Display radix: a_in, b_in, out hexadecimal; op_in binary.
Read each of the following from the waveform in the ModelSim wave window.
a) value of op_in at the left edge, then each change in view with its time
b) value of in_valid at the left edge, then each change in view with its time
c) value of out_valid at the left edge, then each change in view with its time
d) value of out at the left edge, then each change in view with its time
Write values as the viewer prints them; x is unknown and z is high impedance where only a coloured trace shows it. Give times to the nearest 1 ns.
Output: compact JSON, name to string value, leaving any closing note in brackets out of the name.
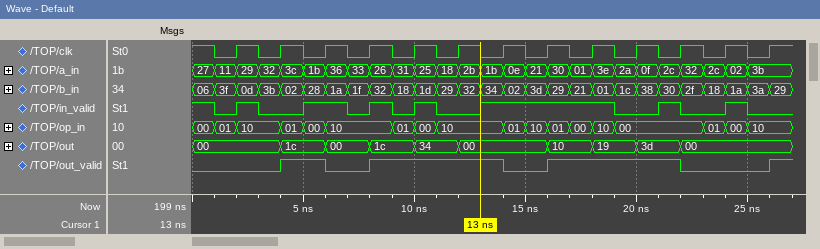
{"value of op_in at the left edge, then each change in view with its time": "00, 01 at 1 ns, 10 at 2 ns, 01 at 4 ns, 00 at 5 ns, 10 at 6 ns, 01 at 9 ns, 00 at 10 ns, 10 at 11 ns, 01 at 14 ns, 10 at 15 ns, 01 at 16 ns, 00 at 17 ns, 10 at 18 ns, 00 at 19 ns, 01 at 23 ns, 00 at 24 ns, 10 at 25 ns", "value of in_valid at the left edge, then each change in view with its time": "1, 0 at 1 ns, 1 at 2 ns, 0 at 3 ns, 1 at 5 ns, 0 at 7 ns, 1 at 8 ns, 0 at 9 ns, 1 at 10 ns, 0 at 11 ns, 1 at 13 ns, 0 at 19 ns, 1 at 21 ns, 0 at 22 ns, 1 at 24 ns, 0 at 25 ns", "value of out_valid at the left edge, then each change in view with its time": "0, 1 at 4 ns, 0 at 6 ns, 1 at 8 ns, 0 at 14 ns, 1 at 16 ns, 0 at 22 ns, 1 at 26 ns", "value of out at the left edge, then each change in view with its time": "00, 1c at 4 ns, 00 at 6 ns, 1c at 8 ns, 34 at 10 ns, 00 at 12 ns, 10 at 16 ns, 19 at 18 ns, 3d at 20 ns, 00 at 22 ns"}
